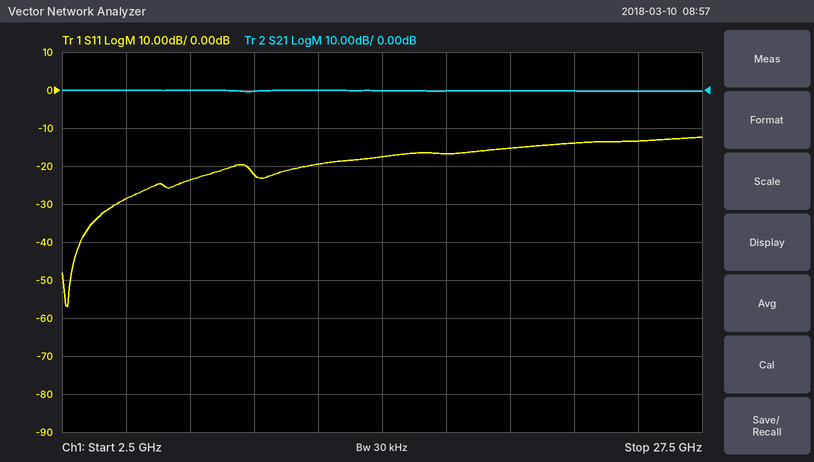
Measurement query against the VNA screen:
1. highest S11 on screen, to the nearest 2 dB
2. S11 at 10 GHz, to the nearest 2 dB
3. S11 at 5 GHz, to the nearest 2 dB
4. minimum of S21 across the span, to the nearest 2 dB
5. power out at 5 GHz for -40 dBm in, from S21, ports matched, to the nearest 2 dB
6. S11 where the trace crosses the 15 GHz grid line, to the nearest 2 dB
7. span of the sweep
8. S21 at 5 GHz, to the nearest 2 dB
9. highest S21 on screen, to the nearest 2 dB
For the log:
-12 dB
-22 dB
-28 dB
0 dB
-40 dBm
-18 dB
25 GHz
0 dB
0 dB
